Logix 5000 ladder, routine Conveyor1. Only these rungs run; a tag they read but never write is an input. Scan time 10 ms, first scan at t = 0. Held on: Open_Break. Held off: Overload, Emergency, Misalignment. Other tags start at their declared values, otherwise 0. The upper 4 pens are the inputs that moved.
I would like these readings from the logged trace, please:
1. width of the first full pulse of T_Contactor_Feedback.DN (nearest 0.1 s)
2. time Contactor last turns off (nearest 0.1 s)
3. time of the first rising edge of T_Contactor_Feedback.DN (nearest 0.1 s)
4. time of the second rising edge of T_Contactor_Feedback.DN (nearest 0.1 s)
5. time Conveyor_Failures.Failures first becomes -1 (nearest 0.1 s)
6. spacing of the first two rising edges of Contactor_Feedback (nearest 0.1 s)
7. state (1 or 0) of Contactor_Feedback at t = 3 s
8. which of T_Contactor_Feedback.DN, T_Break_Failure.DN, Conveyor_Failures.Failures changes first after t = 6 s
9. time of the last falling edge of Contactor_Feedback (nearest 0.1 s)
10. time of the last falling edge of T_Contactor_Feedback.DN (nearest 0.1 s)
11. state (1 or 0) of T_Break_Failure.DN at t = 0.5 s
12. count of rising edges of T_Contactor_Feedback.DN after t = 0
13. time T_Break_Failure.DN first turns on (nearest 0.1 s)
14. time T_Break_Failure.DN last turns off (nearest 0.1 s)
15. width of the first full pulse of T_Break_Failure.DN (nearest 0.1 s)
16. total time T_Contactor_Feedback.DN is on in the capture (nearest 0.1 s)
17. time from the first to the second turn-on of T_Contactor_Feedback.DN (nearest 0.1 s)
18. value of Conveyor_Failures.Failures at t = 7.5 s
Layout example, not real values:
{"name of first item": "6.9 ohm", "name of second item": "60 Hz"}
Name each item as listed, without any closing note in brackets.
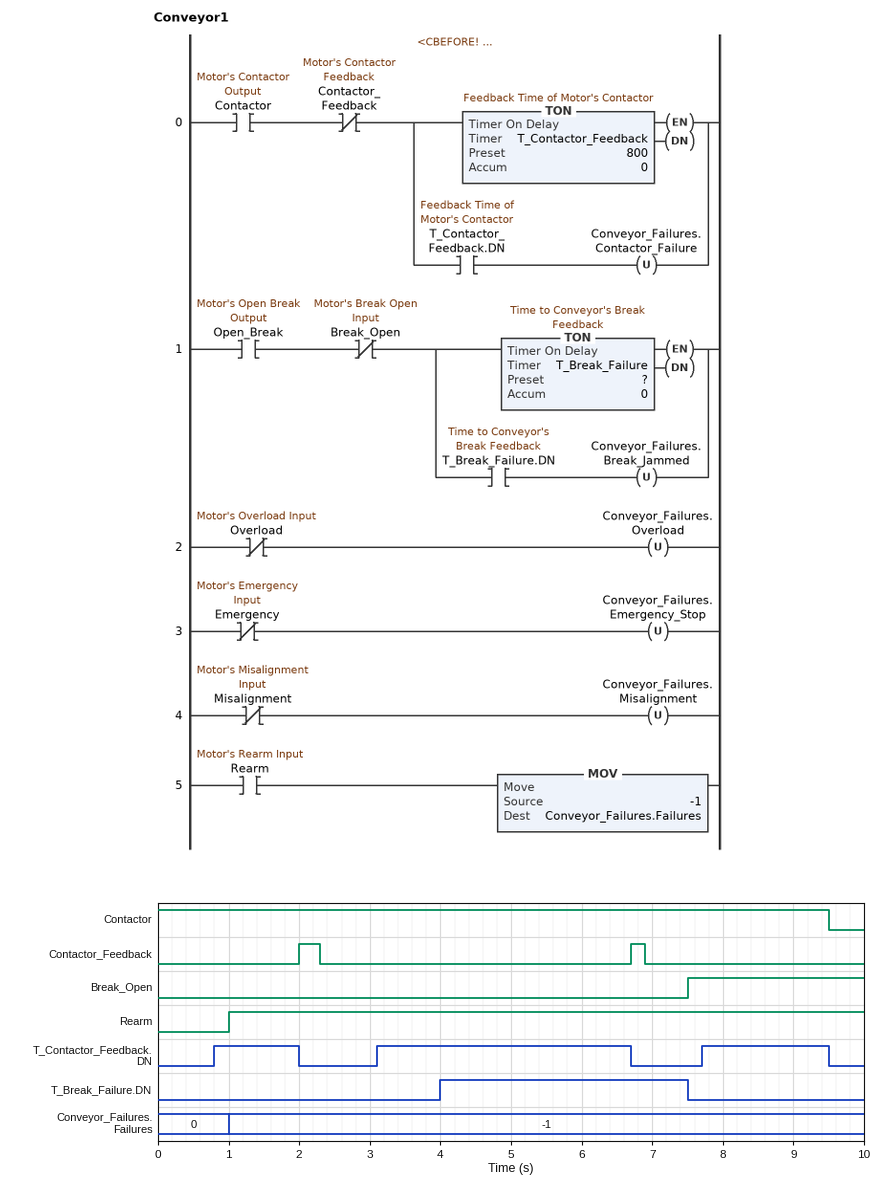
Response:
{"width of the first full pulse of T_Contactor_Feedback.DN": "1.2 s", "time Contactor last turns off": "9.5 s", "time of the first rising edge of T_Contactor_Feedback.DN": "0.8 s", "time of the second rising edge of T_Contactor_Feedback.DN": "3.1 s", "time Conveyor_Failures.Failures first becomes -1": "1.0 s", "spacing of the first two rising edges of Contactor_Feedback": "4.7 s", "state (1 or 0) of Contactor_Feedback at t = 3 s": "0", "which of T_Contactor_Feedback.DN, T_Break_Failure.DN, Conveyor_Failures.Failures changes first after t = 6 s": "T_Contactor_Feedback.DN", "time of the last falling edge of Contactor_Feedback": "6.9 s", "time of the last falling edge of T_Contactor_Feedback.DN": "9.5 s", "state (1 or 0) of T_Break_Failure.DN at t = 0.5 s": "0", "count of rising edges of T_Contactor_Feedback.DN after t = 0": "3", "time T_Break_Failure.DN first turns on": "4.0 s", "time T_Break_Failure.DN last turns off": "7.5 s", "width of the first full pulse of T_Break_Failure.DN": "3.5 s", "total time T_Contactor_Feedback.DN is on in the capture": "6.6 s", "time from the first to the second turn-on of T_Contactor_Feedback.DN": "2.3 s", "value of Conveyor_Failures.Failures at t = 7.5 s": "-1"}
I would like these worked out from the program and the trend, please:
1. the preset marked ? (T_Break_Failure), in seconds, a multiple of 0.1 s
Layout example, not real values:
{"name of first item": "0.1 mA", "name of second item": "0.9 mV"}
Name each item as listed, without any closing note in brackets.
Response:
{"the preset marked ? (T_Break_Failure), in seconds, a multiple of 0.1 s": "4.0 s"}
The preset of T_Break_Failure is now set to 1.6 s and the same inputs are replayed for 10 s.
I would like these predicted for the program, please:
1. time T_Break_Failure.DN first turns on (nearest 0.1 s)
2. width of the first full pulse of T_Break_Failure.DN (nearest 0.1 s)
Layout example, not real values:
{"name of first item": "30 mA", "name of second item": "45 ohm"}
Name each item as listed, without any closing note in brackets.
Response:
{"time T_Break_Failure.DN first turns on": "1.6 s", "width of the first full pulse of T_Break_Failure.DN": "5.9 s"}
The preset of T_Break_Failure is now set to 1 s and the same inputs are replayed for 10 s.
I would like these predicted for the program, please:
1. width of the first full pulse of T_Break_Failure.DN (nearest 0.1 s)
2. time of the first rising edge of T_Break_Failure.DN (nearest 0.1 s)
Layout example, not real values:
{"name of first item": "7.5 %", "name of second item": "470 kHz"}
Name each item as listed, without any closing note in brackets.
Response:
{"width of the first full pulse of T_Break_Failure.DN": "6.5 s", "time of the first rising edge of T_Break_Failure.DN": "1.0 s"}
